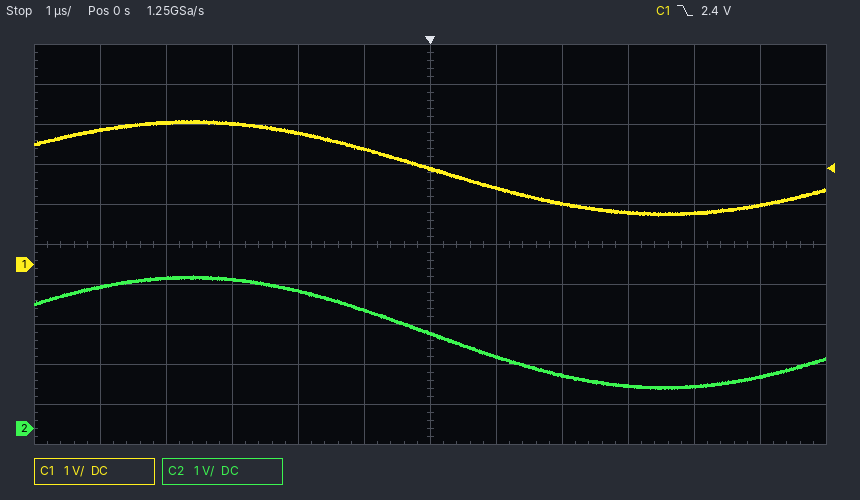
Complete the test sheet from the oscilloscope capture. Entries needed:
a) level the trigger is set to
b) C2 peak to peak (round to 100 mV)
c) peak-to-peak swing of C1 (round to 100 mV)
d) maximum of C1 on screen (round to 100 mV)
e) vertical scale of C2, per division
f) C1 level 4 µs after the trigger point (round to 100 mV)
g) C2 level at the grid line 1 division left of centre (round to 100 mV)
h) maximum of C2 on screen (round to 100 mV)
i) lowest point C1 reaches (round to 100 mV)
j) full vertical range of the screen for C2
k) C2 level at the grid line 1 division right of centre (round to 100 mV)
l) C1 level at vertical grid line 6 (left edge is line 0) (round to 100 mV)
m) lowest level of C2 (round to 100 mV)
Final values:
2.4 V
2.8 V
2.4 V
3.6 V
1 V
1.3 V
3.0 V
3.8 V
1.2 V
10 V
1.8 V
2.4 V
1.0 V
